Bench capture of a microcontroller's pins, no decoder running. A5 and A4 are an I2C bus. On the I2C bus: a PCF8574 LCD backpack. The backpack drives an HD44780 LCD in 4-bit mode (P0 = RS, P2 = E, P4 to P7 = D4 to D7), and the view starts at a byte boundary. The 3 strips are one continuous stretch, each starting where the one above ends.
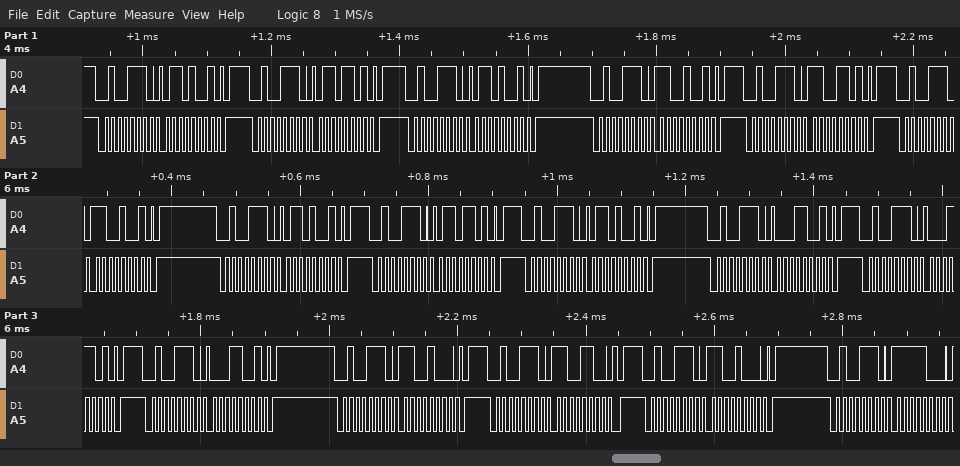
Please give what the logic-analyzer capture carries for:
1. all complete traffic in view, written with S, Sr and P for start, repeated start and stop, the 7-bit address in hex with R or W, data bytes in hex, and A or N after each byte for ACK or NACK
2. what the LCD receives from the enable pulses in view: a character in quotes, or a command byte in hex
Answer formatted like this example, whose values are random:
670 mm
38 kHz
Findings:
S 27W A 69 A P S 27W A 6D A P S 27W A 69 A P S 27W A C9 A P S 27W A CD A P S 27W A C9 A P S 27W A 69 A P S 27W A 6D A P S 27W A 69 A P S 27W A 19 A P S 27W A 1D A P S 27W A 19 A P S 27W A C8 A P S 27W A CC A P S 27W A C8 A P S 27W A F8 A
'l' 'a'
